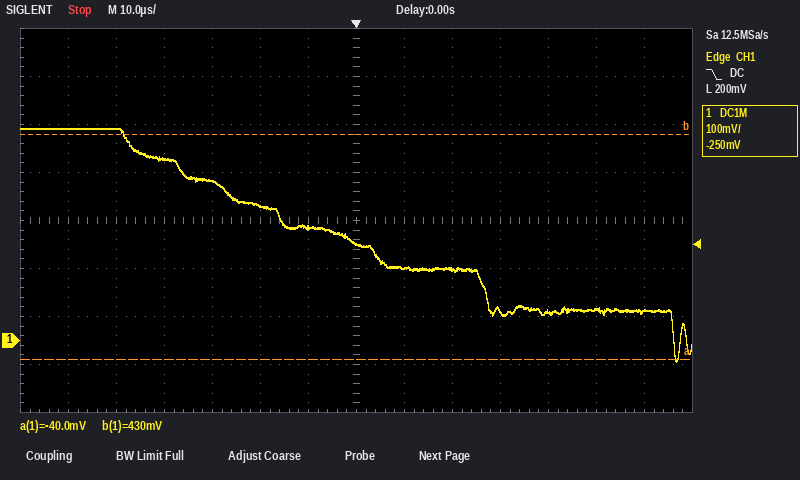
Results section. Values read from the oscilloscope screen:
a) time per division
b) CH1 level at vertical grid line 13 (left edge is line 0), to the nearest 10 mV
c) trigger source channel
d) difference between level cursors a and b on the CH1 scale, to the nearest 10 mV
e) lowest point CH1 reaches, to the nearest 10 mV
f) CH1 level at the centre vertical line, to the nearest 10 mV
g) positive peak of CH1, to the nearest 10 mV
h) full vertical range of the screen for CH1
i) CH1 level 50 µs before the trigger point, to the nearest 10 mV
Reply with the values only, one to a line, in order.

10 µs
60 mV
CH1
470 mV
-40 mV
200 mV
440 mV
800 mV
440 mV
